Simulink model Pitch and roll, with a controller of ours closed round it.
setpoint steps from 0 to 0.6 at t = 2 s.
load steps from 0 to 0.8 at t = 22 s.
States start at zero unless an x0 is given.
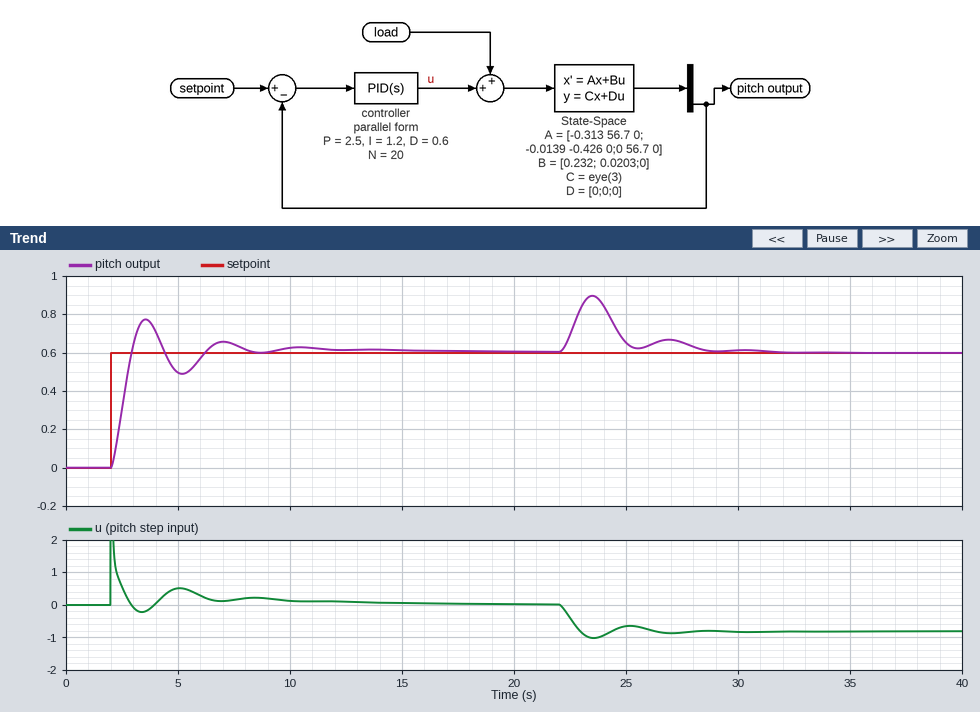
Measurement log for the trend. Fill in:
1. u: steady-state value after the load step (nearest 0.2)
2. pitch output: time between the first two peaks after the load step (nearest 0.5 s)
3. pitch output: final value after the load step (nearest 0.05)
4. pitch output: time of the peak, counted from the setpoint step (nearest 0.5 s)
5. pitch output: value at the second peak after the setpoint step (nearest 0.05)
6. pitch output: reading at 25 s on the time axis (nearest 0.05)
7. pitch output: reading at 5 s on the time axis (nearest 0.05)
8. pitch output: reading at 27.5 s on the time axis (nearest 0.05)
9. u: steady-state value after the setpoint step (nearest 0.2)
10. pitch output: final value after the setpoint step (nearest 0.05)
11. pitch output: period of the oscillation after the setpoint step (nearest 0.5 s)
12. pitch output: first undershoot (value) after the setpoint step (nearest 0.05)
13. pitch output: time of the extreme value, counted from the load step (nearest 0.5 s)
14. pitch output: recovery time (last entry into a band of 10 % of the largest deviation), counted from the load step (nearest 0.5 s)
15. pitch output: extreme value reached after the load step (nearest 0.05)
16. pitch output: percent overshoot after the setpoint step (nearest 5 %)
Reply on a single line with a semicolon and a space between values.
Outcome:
-0.8; 3.5 s; 0.60; 1.5 s; 0.65; 0.65; 0.50; 0.65; 0.0; 0.60; 3.5 s; 0.50; 1.5 s; 6.0 s; 0.90; 30 %
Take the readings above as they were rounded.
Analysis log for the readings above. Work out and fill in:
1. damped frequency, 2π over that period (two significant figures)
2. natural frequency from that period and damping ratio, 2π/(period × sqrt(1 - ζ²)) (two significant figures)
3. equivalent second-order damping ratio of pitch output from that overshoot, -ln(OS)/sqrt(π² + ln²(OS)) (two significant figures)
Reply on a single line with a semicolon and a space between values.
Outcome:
1.8 rad/s; 1.9 rad/s; 0.36
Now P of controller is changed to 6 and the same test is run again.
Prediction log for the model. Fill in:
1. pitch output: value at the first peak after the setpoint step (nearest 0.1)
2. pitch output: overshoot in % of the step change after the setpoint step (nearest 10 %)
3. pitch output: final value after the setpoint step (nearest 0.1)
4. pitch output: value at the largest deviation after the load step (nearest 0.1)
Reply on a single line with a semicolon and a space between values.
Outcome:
0.9; 40 %; 0.6; 0.8
